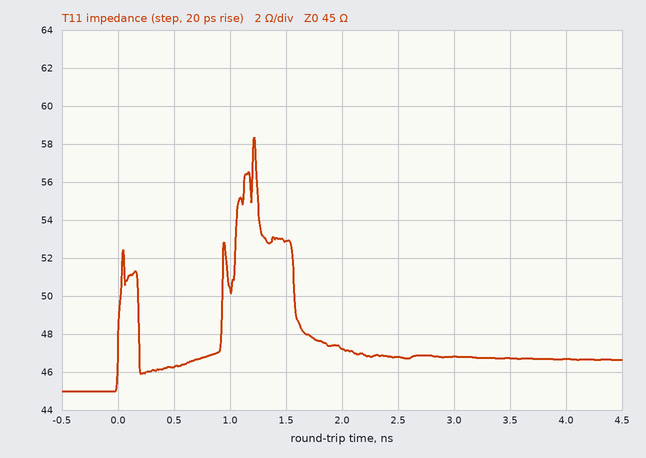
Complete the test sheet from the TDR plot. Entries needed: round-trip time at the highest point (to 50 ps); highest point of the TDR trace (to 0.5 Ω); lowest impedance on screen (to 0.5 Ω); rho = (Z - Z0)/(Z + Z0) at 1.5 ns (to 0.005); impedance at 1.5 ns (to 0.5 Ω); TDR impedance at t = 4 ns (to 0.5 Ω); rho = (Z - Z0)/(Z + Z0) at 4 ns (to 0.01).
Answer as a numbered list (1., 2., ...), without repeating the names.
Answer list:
1. 1.20 ns
2. 58.5 Ω
3. 45.0 Ω
4. +0.080
5. 53.0 Ω
6. 46.5 Ω
7. +0.02
